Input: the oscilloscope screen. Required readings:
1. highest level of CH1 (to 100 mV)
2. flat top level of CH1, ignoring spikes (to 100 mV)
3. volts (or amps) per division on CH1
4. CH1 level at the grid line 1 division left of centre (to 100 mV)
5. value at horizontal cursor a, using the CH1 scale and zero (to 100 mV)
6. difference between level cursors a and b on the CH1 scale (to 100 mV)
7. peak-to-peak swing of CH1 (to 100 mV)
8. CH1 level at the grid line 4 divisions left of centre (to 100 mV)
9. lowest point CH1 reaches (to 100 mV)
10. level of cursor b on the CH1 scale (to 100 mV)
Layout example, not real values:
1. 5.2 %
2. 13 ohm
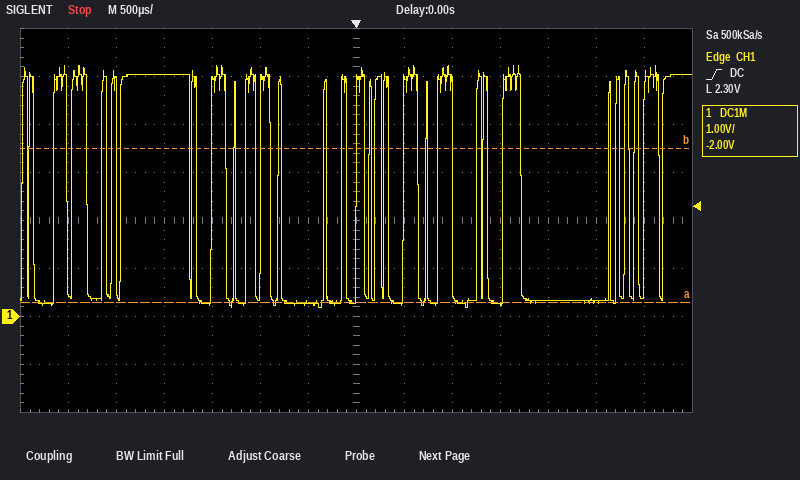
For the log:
1. 5.2 V
2. 5.0 V
3. 1 V
4. 300 mV
5. 300 mV
6. 3.2 V
7. 5.0 V
8. 5.0 V
9. 200 mV
10. 3.5 V
